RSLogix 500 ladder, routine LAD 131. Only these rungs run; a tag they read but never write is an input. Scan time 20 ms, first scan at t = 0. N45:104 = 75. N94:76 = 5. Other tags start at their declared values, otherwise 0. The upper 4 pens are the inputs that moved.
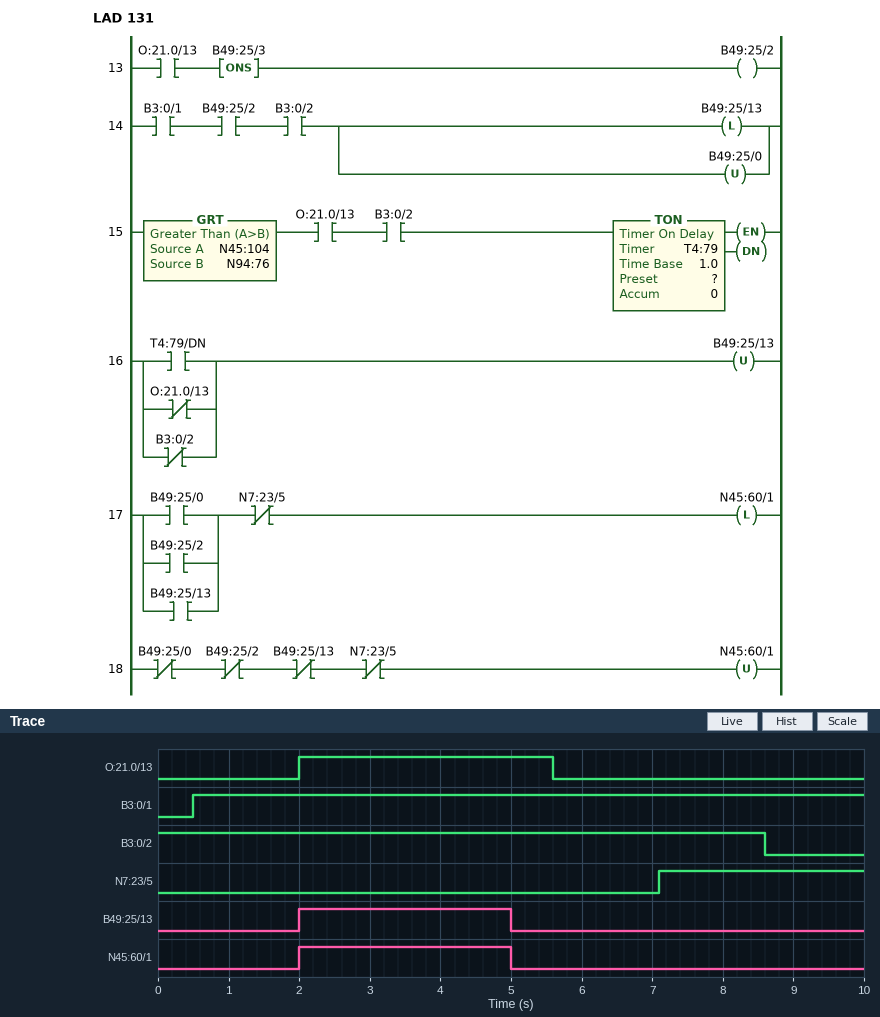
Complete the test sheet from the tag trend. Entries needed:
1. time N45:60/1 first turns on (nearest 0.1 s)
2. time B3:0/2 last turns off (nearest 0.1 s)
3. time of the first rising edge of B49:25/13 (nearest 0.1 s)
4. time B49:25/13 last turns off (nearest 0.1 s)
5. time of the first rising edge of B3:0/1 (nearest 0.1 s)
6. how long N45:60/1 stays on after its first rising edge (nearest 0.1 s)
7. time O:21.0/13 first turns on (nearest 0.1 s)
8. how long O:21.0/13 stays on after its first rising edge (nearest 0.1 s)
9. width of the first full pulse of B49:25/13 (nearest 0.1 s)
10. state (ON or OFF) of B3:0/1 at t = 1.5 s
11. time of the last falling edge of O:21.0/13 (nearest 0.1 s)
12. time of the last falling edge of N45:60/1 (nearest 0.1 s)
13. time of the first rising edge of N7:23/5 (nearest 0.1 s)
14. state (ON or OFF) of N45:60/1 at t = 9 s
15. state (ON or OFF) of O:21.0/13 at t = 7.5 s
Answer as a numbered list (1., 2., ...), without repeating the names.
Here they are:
1. 2.0 s
2. 8.6 s
3. 2.0 s
4. 5.0 s
5. 0.5 s
6. 3.0 s
7. 2.0 s
8. 3.6 s
9. 3.0 s
10. ON
11. 5.6 s
12. 5.0 s
13. 7.1 s
14. OFF
15. OFF
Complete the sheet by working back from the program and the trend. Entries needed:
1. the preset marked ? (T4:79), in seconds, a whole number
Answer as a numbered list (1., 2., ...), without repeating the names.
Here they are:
1. 3 s
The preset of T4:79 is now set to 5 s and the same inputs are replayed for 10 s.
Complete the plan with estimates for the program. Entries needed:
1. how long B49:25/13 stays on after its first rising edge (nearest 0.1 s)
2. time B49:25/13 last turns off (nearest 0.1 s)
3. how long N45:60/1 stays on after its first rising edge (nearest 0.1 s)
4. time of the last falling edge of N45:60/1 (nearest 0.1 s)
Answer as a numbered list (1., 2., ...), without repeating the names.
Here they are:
1. 3.6 s
2. 5.6 s
3. 3.6 s
4. 5.6 s
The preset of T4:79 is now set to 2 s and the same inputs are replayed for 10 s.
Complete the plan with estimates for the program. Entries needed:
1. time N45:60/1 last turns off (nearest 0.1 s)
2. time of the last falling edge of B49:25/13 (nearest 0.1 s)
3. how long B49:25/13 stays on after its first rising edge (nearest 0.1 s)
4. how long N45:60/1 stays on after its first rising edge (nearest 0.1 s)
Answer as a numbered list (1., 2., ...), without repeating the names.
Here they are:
1. 4.0 s
2. 4.0 s
3. 2.0 s
4. 2.0 s
